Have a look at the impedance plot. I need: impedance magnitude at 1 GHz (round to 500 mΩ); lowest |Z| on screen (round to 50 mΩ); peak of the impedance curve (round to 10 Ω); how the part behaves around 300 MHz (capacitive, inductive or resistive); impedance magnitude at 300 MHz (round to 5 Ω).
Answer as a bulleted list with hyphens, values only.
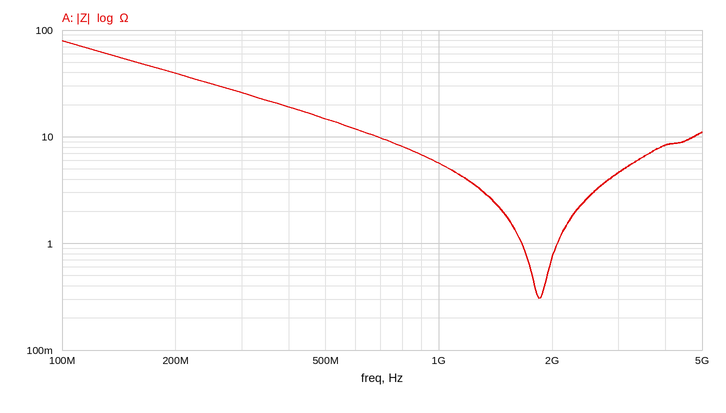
- 5.5 Ω
- 300 mΩ
- 80 Ω
- capacitive
- 25 Ω
